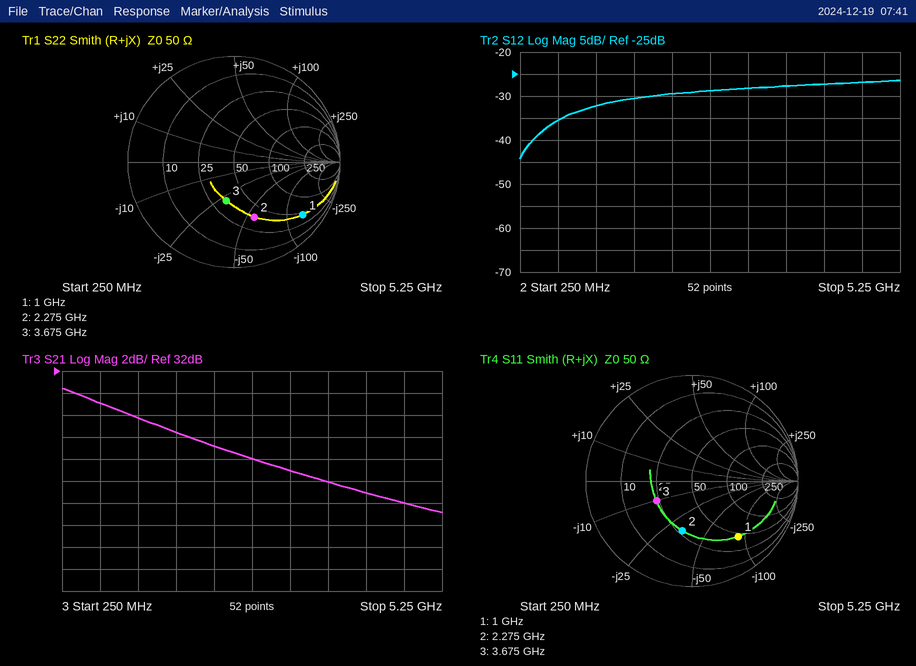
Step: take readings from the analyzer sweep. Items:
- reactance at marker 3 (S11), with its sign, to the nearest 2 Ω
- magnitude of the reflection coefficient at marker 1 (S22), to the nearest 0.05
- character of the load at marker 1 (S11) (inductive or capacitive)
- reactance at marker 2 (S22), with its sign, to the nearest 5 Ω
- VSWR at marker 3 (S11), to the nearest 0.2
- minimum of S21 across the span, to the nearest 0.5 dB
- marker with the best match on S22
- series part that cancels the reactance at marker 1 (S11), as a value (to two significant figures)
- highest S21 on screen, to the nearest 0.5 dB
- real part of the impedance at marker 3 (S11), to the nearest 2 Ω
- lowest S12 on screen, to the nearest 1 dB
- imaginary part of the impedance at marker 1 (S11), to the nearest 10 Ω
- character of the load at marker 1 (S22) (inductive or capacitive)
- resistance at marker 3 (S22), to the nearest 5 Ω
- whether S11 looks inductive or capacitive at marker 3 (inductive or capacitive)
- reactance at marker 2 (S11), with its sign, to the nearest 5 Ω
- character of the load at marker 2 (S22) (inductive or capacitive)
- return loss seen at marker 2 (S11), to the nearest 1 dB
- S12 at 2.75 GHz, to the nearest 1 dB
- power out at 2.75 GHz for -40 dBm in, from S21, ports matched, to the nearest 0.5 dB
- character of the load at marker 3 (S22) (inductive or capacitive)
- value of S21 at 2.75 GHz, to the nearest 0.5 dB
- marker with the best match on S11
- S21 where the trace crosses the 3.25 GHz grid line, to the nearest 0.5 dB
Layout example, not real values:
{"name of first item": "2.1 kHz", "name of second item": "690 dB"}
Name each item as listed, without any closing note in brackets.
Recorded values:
{"reactance at marker 3 (S11), with its sign, to the nearest 2 Ω": "-10 Ω", "magnitude of the reflection coefficient at marker 1 (S22), to the nearest 0.05": "0.80", "character of the load at marker 1 (S11)": "capacitive", "reactance at marker 2 (S22), with its sign, to the nearest 5 Ω": "-55 Ω", "VSWR at marker 3 (S11), to the nearest 0.2": "2.2", "minimum of S21 across the span, to the nearest 0.5 dB": "19.0 dB", "marker with the best match on S22": "marker 3", "series part that cancels the reactance at marker 1 (S11), as a value": "14 nH", "highest S21 on screen, to the nearest 0.5 dB": "30.5 dB", "real part of the impedance at marker 3 (S11), to the nearest 2 Ω": "24 Ω", "lowest S12 on screen, to the nearest 1 dB": "-44 dB", "imaginary part of the impedance at marker 1 (S11), to the nearest 10 Ω": "-90 Ω", "character of the load at marker 1 (S22)": "capacitive", "resistance at marker 3 (S22), to the nearest 5 Ω": "35 Ω", "whether S11 looks inductive or capacitive at marker 3": "capacitive", "reactance at marker 2 (S11), with its sign, to the nearest 5 Ω": "-35 Ω", "character of the load at marker 2 (S22)": "capacitive", "return loss seen at marker 2 (S11), to the nearest 1 dB": "6 dB", "S12 at 2.75 GHz, to the nearest 1 dB": "-29 dB", "power out at 2.75 GHz for -40 dBm in, from S21, ports matched, to the nearest 0.5 dB": "-16.0 dBm", "character of the load at marker 3 (S22)": "capacitive", "value of S21 at 2.75 GHz, to the nearest 0.5 dB": "24.0 dB", "marker with the best match on S11": "marker 3", "S21 where the trace crosses the 3.25 GHz grid line, to the nearest 0.5 dB": "23.0 dB"}
